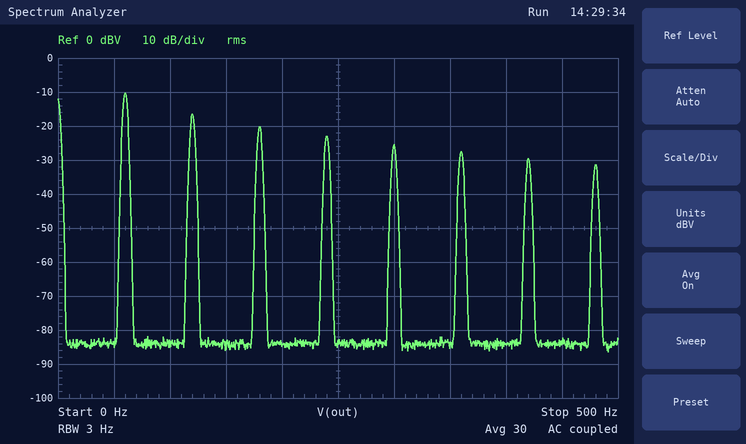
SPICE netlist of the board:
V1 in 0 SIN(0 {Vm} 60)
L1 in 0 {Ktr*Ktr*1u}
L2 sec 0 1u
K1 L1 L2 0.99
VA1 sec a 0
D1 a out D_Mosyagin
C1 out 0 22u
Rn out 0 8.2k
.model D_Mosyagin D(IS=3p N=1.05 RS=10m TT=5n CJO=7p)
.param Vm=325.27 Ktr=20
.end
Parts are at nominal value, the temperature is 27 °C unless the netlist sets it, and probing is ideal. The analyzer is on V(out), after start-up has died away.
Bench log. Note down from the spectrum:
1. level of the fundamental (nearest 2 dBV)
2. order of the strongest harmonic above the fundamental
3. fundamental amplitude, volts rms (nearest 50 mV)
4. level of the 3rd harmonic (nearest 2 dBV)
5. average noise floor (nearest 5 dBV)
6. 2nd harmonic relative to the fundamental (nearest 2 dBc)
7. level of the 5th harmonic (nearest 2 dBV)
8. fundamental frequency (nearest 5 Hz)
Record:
-10 dBV
2
300 mV
-20 dBV
-85 dBV
-6 dBc
-26 dBV
60 Hz
